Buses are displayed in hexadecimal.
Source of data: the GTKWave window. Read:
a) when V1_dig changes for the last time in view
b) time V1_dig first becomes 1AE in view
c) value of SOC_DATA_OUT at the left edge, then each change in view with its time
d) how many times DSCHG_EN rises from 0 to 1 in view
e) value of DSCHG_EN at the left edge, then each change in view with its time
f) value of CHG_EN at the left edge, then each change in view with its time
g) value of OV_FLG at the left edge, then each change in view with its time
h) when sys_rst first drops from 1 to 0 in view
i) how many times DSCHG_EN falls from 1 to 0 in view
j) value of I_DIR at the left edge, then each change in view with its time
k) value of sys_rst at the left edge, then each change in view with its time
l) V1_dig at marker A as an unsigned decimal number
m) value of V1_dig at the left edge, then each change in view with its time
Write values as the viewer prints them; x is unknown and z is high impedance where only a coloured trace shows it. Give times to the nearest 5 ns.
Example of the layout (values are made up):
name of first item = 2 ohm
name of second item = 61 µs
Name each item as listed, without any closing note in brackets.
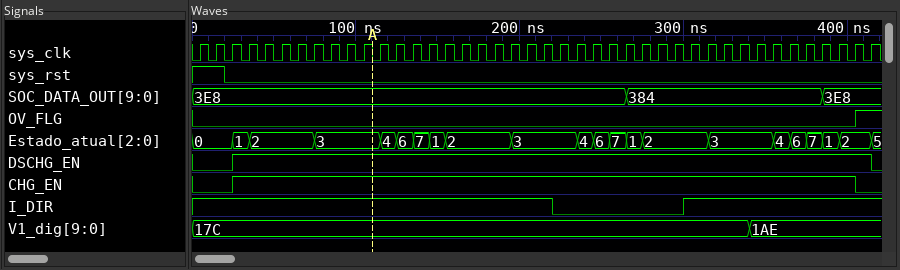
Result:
when V1_dig changes for the last time in view = 340 ns
time V1_dig first becomes 1AE in view = 340 ns
value of SOC_DATA_OUT at the left edge, then each change in view with its time = 3E8, 384 at 265 ns, 3E8 at 385 ns
how many times DSCHG_EN rises from 0 to 1 in view = 1
value of DSCHG_EN at the left edge, then each change in view with its time = 0, 1 at 25 ns, 0 at 415 ns
value of CHG_EN at the left edge, then each change in view with its time = 0, 1 at 25 ns, 0 at 405 ns
value of OV_FLG at the left edge, then each change in view with its time = 0, 1 at 405 ns
when sys_rst first drops from 1 to 0 in view = 20 ns
how many times DSCHG_EN falls from 1 to 0 in view = 1
value of I_DIR at the left edge, then each change in view with its time = 1, 0 at 220 ns, 1 at 300 ns
value of sys_rst at the left edge, then each change in view with its time = 1, 0 at 20 ns
V1_dig at marker A as an unsigned decimal number = 380
value of V1_dig at the left edge, then each change in view with its time = 17C, 1AE at 340 ns
